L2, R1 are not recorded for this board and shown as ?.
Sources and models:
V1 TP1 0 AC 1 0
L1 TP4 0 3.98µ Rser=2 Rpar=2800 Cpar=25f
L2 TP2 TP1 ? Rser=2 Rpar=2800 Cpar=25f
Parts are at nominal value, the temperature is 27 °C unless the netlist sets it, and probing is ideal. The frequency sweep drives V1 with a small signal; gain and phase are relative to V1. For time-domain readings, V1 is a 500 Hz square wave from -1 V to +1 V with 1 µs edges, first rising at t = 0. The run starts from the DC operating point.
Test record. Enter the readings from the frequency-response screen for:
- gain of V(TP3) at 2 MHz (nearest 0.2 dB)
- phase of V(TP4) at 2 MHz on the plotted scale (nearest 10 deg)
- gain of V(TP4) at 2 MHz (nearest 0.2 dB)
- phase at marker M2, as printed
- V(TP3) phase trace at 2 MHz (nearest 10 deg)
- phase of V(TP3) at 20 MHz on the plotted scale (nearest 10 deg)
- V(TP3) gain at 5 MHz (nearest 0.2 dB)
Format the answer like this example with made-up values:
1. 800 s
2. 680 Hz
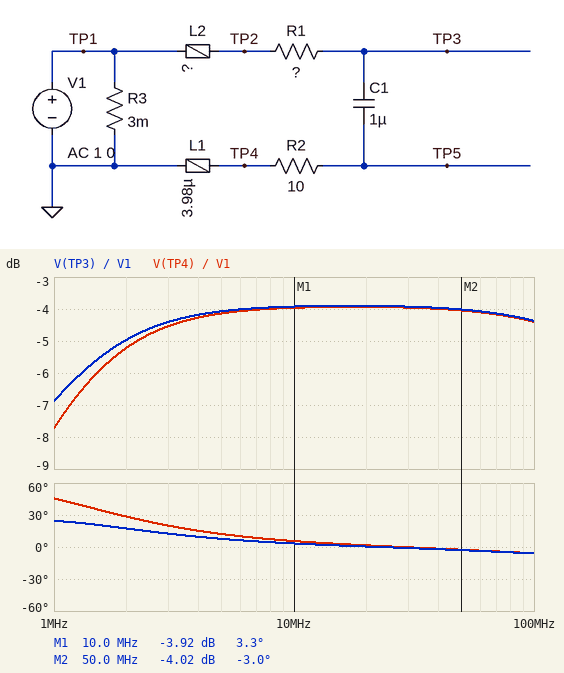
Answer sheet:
1. -5.0 dB
2. 30 deg
3. -5.2 dB
4. -3.0 deg
5. 20 deg
6. 0 deg
7. -4.0 dB
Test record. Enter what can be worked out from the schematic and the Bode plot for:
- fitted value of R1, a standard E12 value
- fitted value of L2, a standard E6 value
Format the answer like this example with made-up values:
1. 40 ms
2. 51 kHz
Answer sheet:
1. 33 Ω
2. 2.2 µH
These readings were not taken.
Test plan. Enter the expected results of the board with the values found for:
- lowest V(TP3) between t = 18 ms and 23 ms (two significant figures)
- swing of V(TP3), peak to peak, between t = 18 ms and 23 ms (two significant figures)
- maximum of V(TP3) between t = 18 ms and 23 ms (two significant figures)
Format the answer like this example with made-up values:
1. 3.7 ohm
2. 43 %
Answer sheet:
1. -1.0 V
2. 2.0 V
3. 1.0 V
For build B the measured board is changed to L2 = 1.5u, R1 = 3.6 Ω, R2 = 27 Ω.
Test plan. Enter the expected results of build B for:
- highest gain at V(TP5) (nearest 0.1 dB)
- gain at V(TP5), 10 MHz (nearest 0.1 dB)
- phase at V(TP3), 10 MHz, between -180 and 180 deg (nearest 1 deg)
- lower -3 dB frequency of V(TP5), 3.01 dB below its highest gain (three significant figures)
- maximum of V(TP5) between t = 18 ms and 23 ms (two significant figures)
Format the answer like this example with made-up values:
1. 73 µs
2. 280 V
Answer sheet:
1. -1.5 dB
2. -2.7 dB
3. -2 deg
4. 4.60 kHz
5. 1.6 V
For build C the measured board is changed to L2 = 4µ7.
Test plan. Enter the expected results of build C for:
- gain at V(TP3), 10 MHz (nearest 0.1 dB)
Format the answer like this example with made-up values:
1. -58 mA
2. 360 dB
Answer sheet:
1. -6.8 dB
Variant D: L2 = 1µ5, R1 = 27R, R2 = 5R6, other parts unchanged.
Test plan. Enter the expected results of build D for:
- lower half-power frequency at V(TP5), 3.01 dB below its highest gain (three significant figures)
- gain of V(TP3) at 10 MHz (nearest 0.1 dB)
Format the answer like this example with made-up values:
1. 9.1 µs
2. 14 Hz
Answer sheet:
1. 953 kHz
2. -2.9 dB
